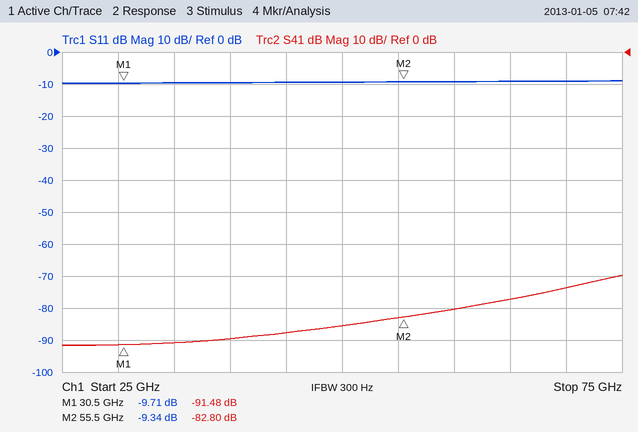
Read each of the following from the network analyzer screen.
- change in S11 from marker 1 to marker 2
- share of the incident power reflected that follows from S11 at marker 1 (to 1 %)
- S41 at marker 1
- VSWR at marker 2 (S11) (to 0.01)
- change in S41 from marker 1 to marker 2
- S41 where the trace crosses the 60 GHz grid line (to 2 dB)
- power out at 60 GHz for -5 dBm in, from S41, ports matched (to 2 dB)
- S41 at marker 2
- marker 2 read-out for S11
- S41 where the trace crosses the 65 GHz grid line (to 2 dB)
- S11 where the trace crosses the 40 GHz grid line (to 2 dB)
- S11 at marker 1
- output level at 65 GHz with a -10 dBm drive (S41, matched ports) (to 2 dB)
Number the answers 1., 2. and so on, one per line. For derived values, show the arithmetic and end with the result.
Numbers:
1. -9.34 − (-9.71) = 0.37 dB
2. 10^(-9.71/10) ≈ 11 %
3. -91.48 dB
4. (1 + 0.3412)/(1 − 0.3412) ≈ 2.04
5. -82.8 − (-91.48) = 8.68 dB
6. -80 dB
7. -5 dBm + (-80 dB) = -86 dBm
8. -82.80 dB
9. -9.34 dB
10. -78 dB
11. -10 dB
12. -9.71 dB
13. -10 dBm + (-78 dB) = -88 dBm
